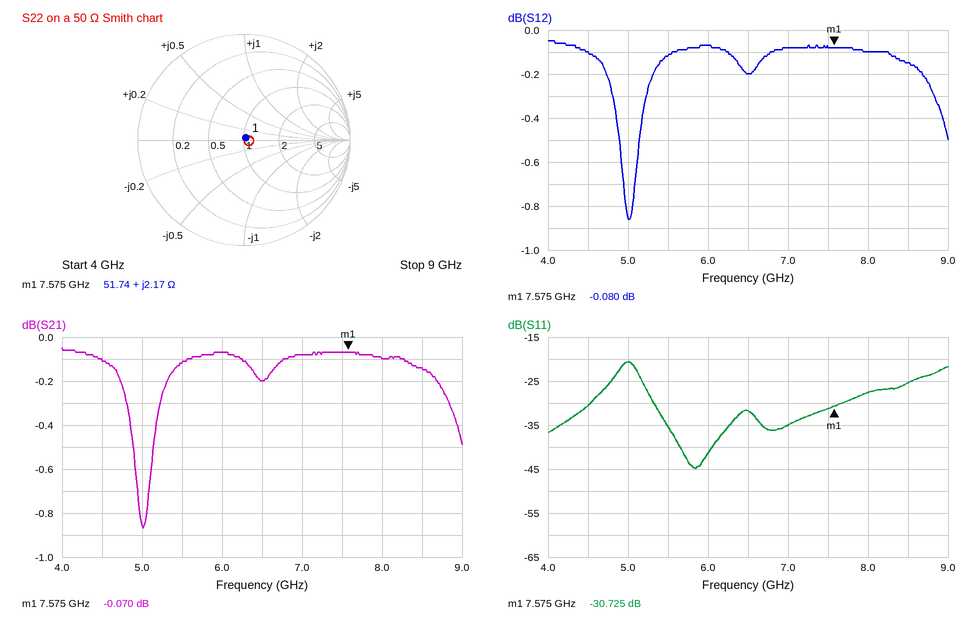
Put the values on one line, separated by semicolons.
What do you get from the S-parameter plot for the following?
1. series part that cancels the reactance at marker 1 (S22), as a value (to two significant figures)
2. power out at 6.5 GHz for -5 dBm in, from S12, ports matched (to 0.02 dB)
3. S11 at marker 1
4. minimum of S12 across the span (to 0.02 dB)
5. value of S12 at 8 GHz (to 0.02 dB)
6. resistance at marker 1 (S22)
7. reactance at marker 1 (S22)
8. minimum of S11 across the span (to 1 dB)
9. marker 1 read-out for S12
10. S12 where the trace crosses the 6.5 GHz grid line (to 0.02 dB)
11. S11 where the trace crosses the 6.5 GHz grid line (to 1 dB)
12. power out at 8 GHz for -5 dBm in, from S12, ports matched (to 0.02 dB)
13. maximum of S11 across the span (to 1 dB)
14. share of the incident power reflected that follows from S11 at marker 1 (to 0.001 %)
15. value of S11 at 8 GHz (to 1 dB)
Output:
9.7 pF; -5.20 dBm; -30.725 dB; -0.86 dB; -0.10 dB; 51.74 Ω; +2.17 Ω; -45 dB; -0.080 dB; -0.20 dB; -32 dB; -5.10 dBm; -21 dB; 0.085 %; -28 dB
